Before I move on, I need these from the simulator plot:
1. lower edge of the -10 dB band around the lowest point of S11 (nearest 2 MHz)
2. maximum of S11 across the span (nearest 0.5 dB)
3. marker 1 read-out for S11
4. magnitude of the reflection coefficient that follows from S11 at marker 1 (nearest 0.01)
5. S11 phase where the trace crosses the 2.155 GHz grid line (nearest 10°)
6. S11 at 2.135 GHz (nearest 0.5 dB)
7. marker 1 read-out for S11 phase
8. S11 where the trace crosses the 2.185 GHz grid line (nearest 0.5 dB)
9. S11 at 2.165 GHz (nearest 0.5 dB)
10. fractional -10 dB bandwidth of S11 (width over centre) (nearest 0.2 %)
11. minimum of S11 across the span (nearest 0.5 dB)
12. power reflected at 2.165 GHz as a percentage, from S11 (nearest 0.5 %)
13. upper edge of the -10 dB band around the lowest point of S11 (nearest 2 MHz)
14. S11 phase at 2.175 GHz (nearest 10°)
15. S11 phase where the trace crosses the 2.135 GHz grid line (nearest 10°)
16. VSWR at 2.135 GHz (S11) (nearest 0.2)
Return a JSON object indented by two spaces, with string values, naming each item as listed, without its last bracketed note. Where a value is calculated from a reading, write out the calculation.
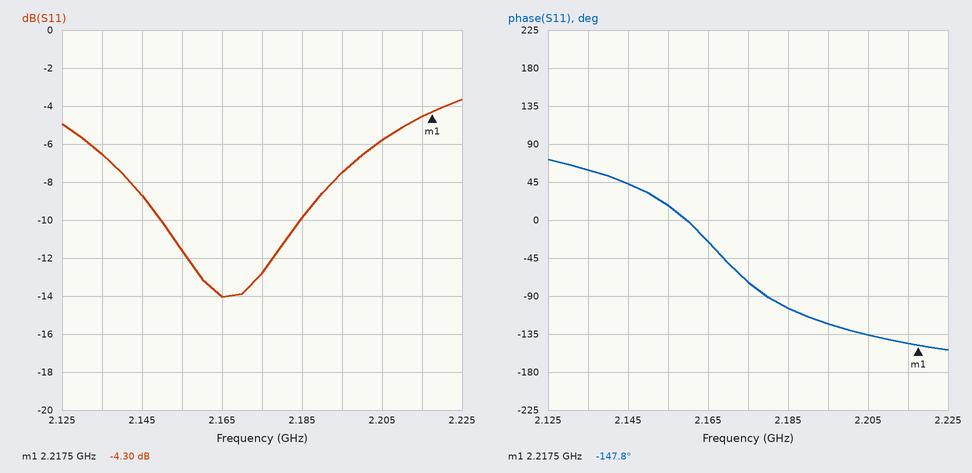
{
  "lower edge of the -10 dB band around the lowest point of S11": "2.150 GHz",
  "maximum of S11 across the span": "-3.5 dB",
  "marker 1 read-out for S11": "-4.30 dB",
  "magnitude of the reflection coefficient that follows from S11 at marker 1": "10^(-4.3/20) ≈ 0.61",
  "S11 phase where the trace crosses the 2.155 GHz grid line": "20°",
  "S11 at 2.135 GHz": "-6.5 dB",
  "marker 1 read-out for S11 phase": "-147.8°",
  "S11 where the trace crosses the 2.185 GHz grid line": "-10.0 dB",
  "S11 at 2.165 GHz": "-14.0 dB",
  "fractional -10 dB bandwidth of S11 (width over centre)": "34 MHz / 2.167 GHz ≈ 1.6 %",
  "minimum of S11 across the span": "-14.0 dB",
  "power reflected at 2.165 GHz as a percentage, from S11": "10^(-14/10) ≈ 4.0 %",
  "upper edge of the -10 dB band around the lowest point of S11": "2.184 GHz",
  "S11 phase at 2.175 GHz": "-70°",
  "S11 phase where the trace crosses the 2.135 GHz grid line": "60°",
  "VSWR at 2.135 GHz (S11)": "|Γ| = 10^(-6.5/20) = 0.4732; VSWR = (1 + 0.4732)/(1 − 0.4732) ≈ 2.8"
}
